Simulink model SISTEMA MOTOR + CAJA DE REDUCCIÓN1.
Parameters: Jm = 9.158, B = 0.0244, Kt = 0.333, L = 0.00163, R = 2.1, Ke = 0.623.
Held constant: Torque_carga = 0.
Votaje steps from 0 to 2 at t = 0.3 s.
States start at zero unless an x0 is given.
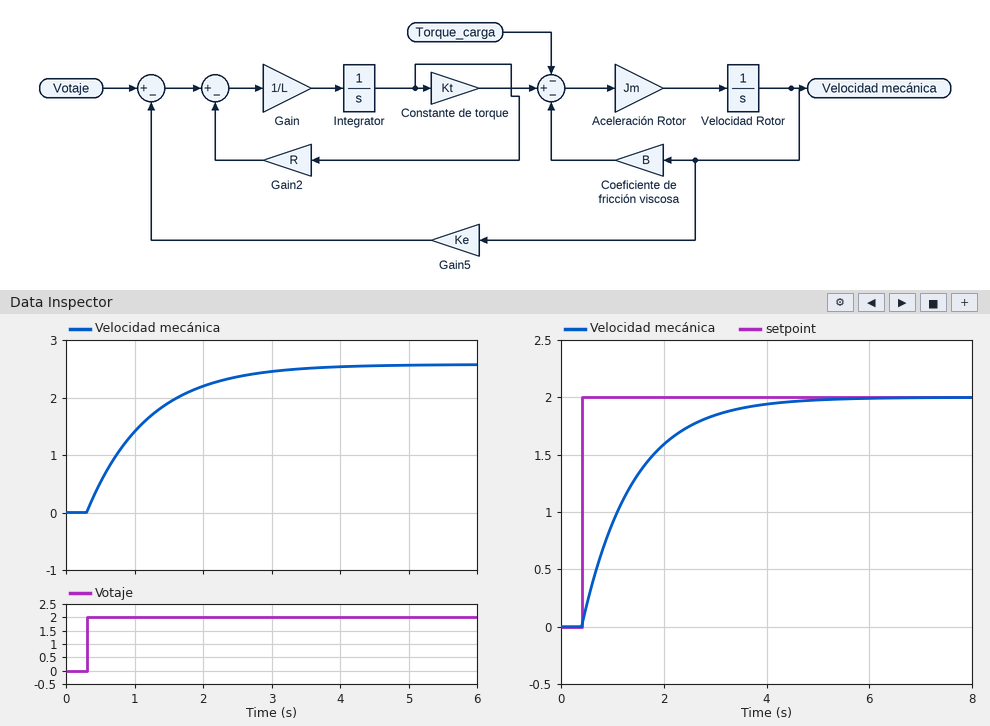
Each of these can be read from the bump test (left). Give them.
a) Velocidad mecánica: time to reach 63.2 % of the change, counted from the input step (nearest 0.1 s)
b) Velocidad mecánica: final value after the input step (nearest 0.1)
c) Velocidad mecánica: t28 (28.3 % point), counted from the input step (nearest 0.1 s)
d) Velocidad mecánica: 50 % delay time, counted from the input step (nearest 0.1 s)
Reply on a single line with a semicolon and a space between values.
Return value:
0.9 s; 2.6; 0.3 s; 0.6 s
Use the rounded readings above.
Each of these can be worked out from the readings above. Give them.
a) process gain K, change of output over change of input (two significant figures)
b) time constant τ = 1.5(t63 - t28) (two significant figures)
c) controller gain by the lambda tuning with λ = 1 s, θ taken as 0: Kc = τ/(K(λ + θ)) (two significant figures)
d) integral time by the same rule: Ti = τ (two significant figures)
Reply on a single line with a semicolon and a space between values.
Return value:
1.3; 0.90 s; 0.69; 0.90 s
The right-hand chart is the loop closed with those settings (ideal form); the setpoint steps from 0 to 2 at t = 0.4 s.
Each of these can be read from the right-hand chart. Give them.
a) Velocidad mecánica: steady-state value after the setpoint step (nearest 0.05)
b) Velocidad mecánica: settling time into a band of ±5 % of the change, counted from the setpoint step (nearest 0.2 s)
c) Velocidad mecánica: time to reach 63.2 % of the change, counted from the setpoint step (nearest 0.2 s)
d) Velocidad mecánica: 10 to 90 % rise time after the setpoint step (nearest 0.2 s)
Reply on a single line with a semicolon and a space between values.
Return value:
2.00; 3.0 s; 1.0 s; 2.2 s
